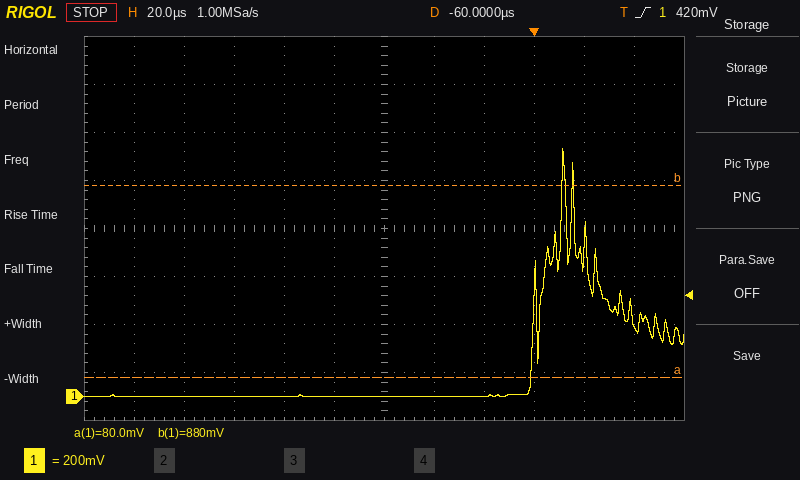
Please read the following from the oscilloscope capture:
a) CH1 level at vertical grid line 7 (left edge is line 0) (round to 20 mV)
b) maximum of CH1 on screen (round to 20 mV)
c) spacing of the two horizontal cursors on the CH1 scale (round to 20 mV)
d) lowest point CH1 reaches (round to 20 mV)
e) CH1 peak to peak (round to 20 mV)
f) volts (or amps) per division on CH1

0 mV
1.04 V
800 mV
0 mV
1.04 V
200 mV
